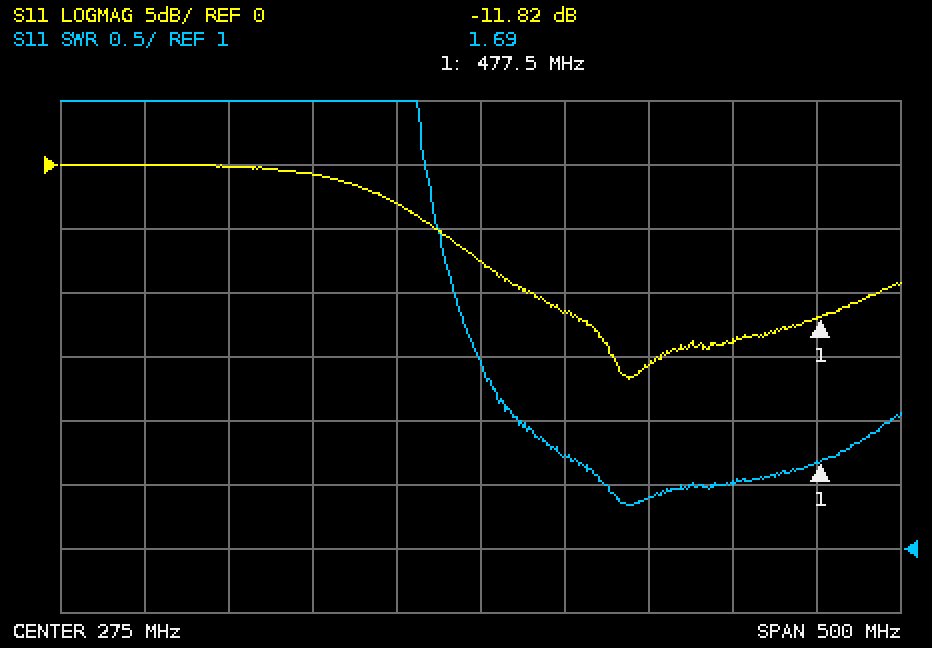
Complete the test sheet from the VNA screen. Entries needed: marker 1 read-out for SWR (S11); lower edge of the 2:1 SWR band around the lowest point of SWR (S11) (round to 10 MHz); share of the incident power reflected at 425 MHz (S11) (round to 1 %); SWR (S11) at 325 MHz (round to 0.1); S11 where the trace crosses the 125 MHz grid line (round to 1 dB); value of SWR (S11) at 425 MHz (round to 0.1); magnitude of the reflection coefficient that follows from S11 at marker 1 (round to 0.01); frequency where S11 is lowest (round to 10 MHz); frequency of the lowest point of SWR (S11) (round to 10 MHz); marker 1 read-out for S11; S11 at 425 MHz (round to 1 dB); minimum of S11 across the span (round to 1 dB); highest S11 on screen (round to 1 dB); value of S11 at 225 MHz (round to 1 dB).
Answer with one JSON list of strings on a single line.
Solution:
["1.69", "300 MHz", "4 %", "1.7", "0 dB", "1.5", "0.26", "360 MHz", "360 MHz", "-11.82 dB", "-14 dB", "-17 dB", "0 dB", "-3 dB"]
